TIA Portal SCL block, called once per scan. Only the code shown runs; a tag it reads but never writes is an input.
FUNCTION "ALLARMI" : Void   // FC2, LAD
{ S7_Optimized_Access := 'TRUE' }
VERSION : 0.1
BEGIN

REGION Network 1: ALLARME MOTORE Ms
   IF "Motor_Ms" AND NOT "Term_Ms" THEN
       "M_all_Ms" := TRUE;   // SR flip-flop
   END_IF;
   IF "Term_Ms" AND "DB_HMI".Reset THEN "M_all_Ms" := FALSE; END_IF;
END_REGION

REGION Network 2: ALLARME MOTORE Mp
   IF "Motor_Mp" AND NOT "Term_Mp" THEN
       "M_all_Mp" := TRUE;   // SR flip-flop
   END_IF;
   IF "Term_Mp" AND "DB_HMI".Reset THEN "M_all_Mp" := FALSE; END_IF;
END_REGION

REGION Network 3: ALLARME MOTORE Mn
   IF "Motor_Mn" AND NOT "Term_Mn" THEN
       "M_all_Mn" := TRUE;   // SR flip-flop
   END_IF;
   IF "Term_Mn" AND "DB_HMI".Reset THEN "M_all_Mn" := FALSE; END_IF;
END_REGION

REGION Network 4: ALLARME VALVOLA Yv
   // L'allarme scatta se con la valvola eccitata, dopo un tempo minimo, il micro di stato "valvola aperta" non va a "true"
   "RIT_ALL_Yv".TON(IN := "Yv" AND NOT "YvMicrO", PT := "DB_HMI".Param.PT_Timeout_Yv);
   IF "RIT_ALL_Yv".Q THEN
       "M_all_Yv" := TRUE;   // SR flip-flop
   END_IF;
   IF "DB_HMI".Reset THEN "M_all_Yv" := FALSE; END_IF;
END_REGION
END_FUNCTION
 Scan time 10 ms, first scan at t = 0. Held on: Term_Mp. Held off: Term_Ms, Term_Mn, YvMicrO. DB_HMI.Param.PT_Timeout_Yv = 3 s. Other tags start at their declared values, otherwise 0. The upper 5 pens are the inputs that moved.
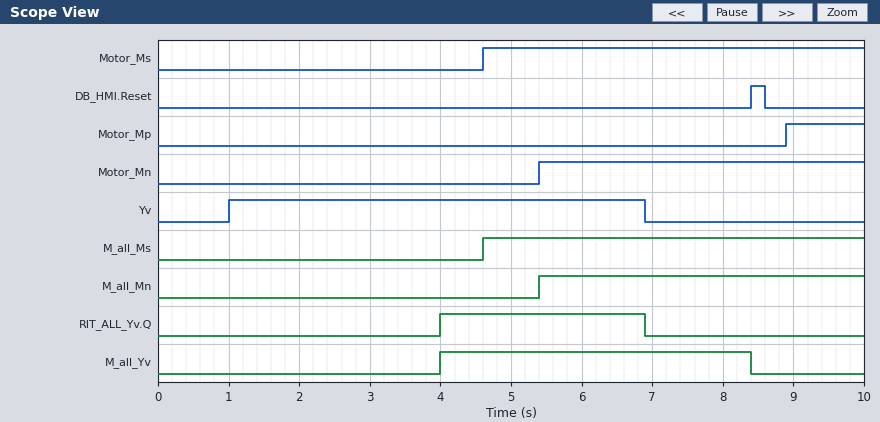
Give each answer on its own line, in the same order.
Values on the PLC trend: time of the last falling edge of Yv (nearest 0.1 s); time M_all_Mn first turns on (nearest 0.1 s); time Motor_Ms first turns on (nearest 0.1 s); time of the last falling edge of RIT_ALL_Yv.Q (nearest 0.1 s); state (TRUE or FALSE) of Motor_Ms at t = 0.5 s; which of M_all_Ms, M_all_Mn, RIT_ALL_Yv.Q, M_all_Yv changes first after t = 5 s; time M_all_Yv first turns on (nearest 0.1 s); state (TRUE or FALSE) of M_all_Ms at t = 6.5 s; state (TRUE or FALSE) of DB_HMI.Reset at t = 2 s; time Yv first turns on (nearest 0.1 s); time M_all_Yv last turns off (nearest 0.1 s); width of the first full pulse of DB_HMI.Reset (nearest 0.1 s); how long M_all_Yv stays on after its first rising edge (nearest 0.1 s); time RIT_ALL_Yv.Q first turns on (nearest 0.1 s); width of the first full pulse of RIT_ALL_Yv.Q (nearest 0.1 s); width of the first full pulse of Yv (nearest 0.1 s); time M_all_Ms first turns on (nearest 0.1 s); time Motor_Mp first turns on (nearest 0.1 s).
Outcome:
6.9 s
5.4 s
4.6 s
6.9 s
FALSE
M_all_Mn
4.0 s
TRUE
FALSE
1.0 s
8.4 s
0.2 s
4.4 s
4.0 s
2.9 s
5.9 s
4.6 s
8.9 s
